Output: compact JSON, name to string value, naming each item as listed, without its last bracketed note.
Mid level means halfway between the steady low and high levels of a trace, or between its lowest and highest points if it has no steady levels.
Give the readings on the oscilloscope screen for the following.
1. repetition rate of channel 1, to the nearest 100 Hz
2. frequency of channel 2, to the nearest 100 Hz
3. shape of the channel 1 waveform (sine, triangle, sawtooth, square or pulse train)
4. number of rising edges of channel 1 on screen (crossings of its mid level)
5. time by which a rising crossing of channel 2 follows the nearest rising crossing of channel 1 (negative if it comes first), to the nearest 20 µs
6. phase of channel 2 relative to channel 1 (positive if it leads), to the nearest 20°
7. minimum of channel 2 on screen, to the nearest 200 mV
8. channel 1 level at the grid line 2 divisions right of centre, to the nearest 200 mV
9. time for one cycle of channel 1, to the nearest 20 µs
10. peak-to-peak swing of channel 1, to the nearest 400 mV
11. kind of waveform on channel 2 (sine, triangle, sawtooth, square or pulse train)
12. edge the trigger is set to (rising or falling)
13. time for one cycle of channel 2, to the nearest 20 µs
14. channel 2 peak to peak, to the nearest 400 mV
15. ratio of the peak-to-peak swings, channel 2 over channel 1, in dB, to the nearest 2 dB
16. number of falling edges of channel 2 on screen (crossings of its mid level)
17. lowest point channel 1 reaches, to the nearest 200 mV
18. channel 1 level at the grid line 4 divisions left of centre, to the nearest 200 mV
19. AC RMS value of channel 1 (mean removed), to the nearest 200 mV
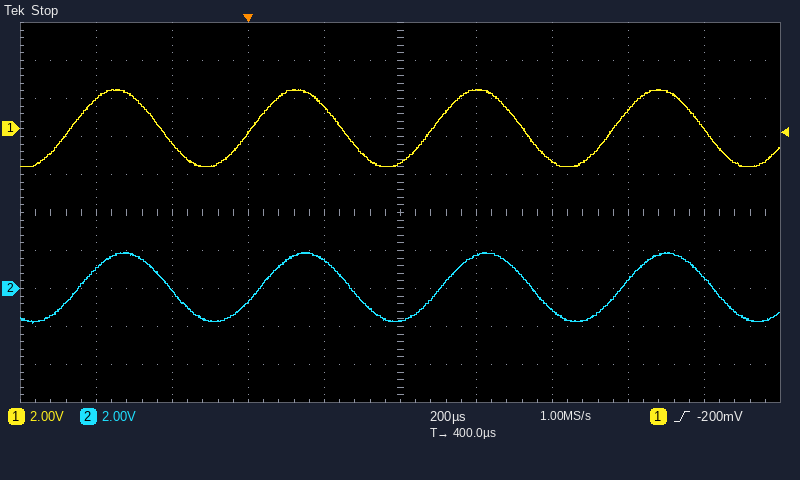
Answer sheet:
{"repetition rate of channel 1, to the nearest 100 Hz": "2.1 kHz", "frequency of channel 2, to the nearest 100 Hz": "2.1 kHz", "shape of the channel 1 waveform": "sine", "number of rising edges of channel 1 on screen": "4", "time by which a rising crossing of channel 2 follows the nearest rising crossing of channel 1 (negative if it comes first), to the nearest 20 µs": "+20 µs", "phase of channel 2 relative to channel 1 (positive if it leads), to the nearest 20°": "-20°", "minimum of channel 2 on screen, to the nearest 200 mV": "-1.8 V", "channel 1 level at the grid line 2 divisions right of centre, to the nearest 200 mV": "-1.6 V", "time for one cycle of channel 1, to the nearest 20 µs": "480 µs", "peak-to-peak swing of channel 1, to the nearest 400 mV": "4.0 V", "kind of waveform on channel 2": "sine", "edge the trigger is set to": "rising", "time for one cycle of channel 2, to the nearest 20 µs": "480 µs", "channel 2 peak to peak, to the nearest 400 mV": "3.6 V", "ratio of the peak-to-peak swings, channel 2 over channel 1, in dB, to the nearest 2 dB": "0 dB", "number of falling edges of channel 2 on screen": "4", "lowest point channel 1 reaches, to the nearest 200 mV": "-2.0 V", "channel 1 level at the grid line 4 divisions left of centre, to the nearest 200 mV": "1.6 V", "AC RMS value of channel 1 (mean removed), to the nearest 200 mV": "1.4 V"}
